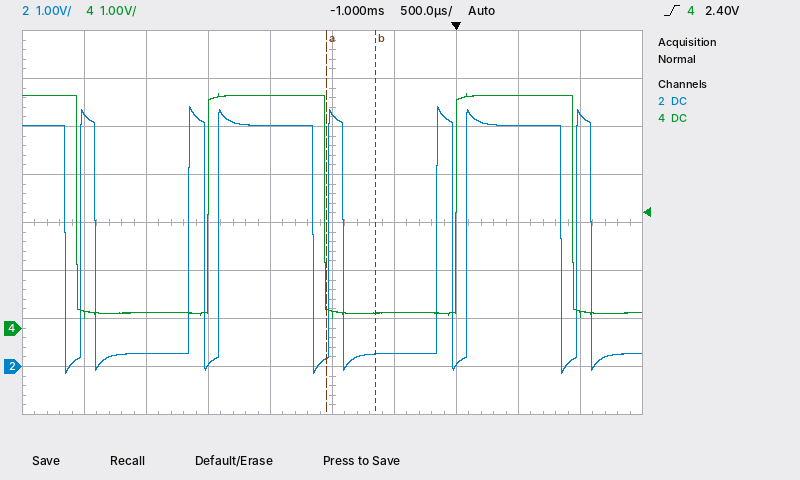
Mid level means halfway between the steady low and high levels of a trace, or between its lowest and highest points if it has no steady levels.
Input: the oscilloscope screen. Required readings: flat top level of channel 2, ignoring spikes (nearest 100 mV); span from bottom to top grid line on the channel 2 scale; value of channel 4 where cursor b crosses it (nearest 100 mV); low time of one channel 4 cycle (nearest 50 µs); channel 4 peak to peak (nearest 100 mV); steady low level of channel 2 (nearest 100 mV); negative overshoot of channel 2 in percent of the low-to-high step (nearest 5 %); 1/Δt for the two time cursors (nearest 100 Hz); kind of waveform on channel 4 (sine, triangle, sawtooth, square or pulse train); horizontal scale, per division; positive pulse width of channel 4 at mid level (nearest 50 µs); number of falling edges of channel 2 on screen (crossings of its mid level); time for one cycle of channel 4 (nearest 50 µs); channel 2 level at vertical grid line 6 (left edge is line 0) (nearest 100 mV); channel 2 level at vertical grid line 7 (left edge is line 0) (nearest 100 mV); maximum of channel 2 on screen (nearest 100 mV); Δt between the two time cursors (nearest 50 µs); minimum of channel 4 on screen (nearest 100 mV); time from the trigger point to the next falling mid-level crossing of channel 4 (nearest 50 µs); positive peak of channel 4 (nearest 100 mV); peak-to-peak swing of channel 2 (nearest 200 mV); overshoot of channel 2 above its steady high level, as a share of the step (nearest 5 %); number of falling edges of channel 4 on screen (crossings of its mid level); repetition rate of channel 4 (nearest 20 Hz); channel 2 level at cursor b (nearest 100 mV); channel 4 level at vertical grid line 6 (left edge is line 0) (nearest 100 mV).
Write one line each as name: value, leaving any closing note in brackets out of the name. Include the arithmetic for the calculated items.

flat top level of channel 2, ignoring spikes: 5.0 V
span from bottom to top grid line on the channel 2 scale: 8 V
value of channel 4 where cursor b crosses it: 300 mV
low time of one channel 4 cycle: 1.05 ms
channel 4 peak to peak: 4.9 V − (200 mV) = 4.7 V
steady low level of channel 2: 300 mV
negative overshoot of channel 2 in percent of the low-to-high step: 10 %
1/Δt for the two time cursors: 1 / 400 µs ≈ 2.5 kHz
kind of waveform on channel 4: square
horizontal scale, per division: 500 µs
positive pulse width of channel 4 at mid level: 950 µs
number of falling edges of channel 2 on screen: 8
time for one cycle of channel 4: 2.00 ms
channel 2 level at vertical grid line 6 (left edge is line 0): 300 mV
channel 2 level at vertical grid line 7 (left edge is line 0): 0.0 V
maximum of channel 2 on screen: 5.4 V
Δt between the two time cursors: 400 µs
minimum of channel 4 on screen: 200 mV
time from the trigger point to the next falling mid-level crossing of channel 4: 950 µs
positive peak of channel 4: 4.9 V
peak-to-peak swing of channel 2: 5.6 V
overshoot of channel 2 above its steady high level, as a share of the step: 10 %
number of falling edges of channel 4 on screen: 3
repetition rate of channel 4: 1 / 2.00 ms ≈ 500 Hz
channel 2 level at cursor b: 300 mV
channel 4 level at vertical grid line 6 (left edge is line 0): 300 mV
